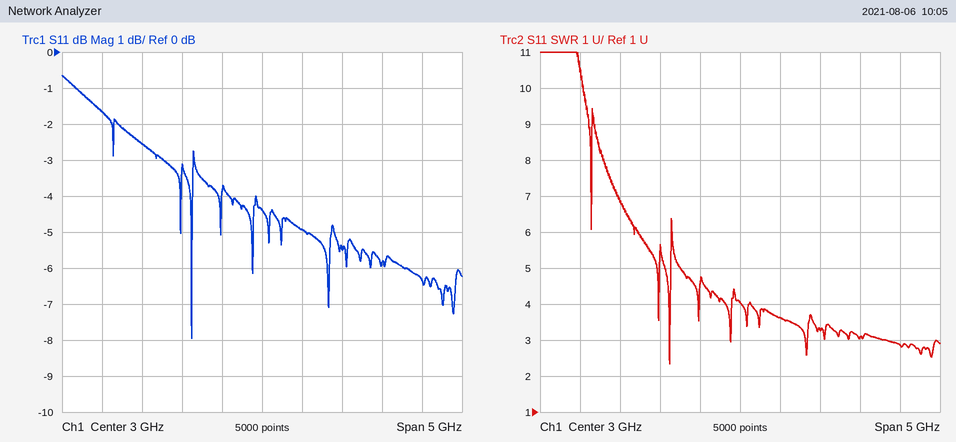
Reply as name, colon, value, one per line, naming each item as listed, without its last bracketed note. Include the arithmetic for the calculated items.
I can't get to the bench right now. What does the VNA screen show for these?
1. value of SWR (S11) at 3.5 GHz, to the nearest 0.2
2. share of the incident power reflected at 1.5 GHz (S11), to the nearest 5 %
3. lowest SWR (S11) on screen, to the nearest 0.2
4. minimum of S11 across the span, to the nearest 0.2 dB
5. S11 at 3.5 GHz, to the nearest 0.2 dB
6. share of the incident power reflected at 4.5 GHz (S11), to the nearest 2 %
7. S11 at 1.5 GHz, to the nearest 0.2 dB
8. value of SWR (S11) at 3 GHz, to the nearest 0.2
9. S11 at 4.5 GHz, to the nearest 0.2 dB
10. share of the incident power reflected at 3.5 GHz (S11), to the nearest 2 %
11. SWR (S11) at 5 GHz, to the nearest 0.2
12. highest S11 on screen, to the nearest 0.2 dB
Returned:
value of SWR (S11) at 3.5 GHz, to the nearest 0.2: 3.6
share of the incident power reflected at 1.5 GHz (S11), to the nearest 5 %: 10^(-2.6/10) ≈ 55 %
lowest SWR (S11) on screen, to the nearest 0.2: 2.4
minimum of S11 across the span, to the nearest 0.2 dB: -8.0 dB
S11 at 3.5 GHz, to the nearest 0.2 dB: -5.0 dB
share of the incident power reflected at 4.5 GHz (S11), to the nearest 2 %: 10^(-5.8/10) ≈ 26 %
S11 at 1.5 GHz, to the nearest 0.2 dB: -2.6 dB
value of SWR (S11) at 3 GHz, to the nearest 0.2: 4.0
S11 at 4.5 GHz, to the nearest 0.2 dB: -5.8 dB
share of the incident power reflected at 3.5 GHz (S11), to the nearest 2 %: 10^(-5/10) ≈ 32 %
SWR (S11) at 5 GHz, to the nearest 0.2: 2.8
highest S11 on screen, to the nearest 0.2 dB: -0.6 dB
